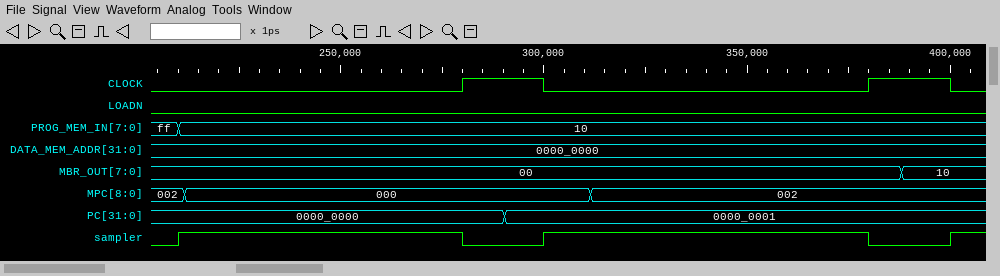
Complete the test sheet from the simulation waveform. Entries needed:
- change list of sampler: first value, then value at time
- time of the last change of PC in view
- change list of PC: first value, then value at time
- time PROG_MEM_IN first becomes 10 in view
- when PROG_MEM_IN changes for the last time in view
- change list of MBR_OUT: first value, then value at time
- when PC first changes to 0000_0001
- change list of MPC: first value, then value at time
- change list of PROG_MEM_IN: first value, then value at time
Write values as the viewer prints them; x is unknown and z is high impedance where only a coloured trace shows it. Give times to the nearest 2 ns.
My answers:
0, 1 at 210 ns, 0 at 280 ns, 1 at 300 ns, 0 at 380 ns, 1 at 400 ns
290 ns
0000_0000, 0000_0001 at 290 ns
210 ns
210 ns
00, 10 at 388 ns
290 ns
002, 000 at 212 ns, 002 at 312 ns
ff, 10 at 210 ns
